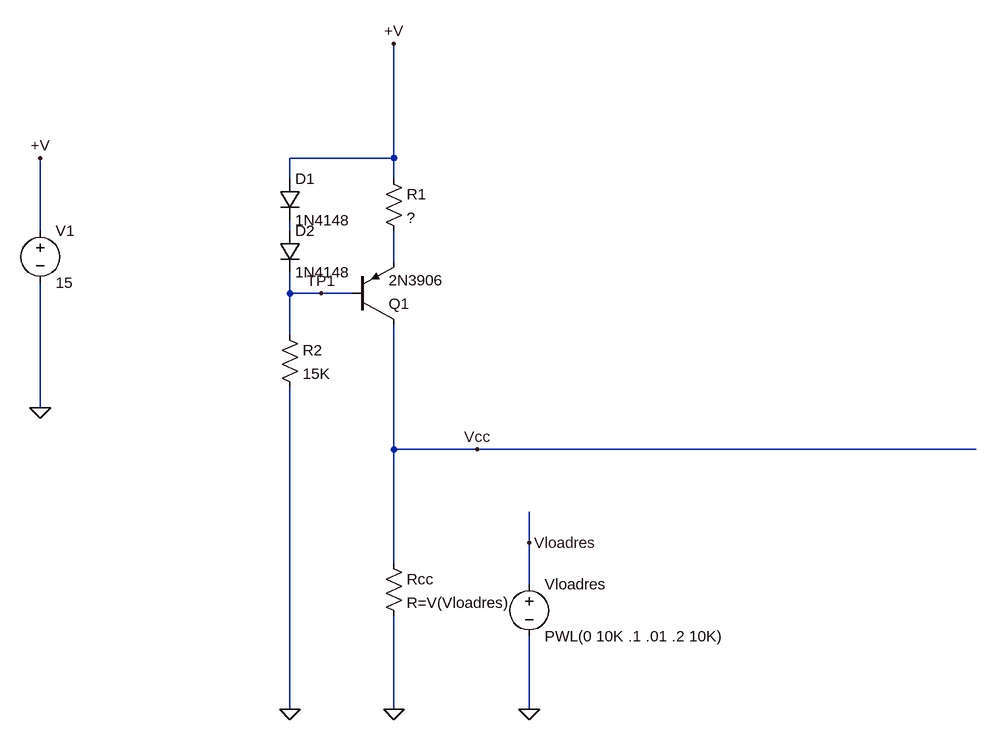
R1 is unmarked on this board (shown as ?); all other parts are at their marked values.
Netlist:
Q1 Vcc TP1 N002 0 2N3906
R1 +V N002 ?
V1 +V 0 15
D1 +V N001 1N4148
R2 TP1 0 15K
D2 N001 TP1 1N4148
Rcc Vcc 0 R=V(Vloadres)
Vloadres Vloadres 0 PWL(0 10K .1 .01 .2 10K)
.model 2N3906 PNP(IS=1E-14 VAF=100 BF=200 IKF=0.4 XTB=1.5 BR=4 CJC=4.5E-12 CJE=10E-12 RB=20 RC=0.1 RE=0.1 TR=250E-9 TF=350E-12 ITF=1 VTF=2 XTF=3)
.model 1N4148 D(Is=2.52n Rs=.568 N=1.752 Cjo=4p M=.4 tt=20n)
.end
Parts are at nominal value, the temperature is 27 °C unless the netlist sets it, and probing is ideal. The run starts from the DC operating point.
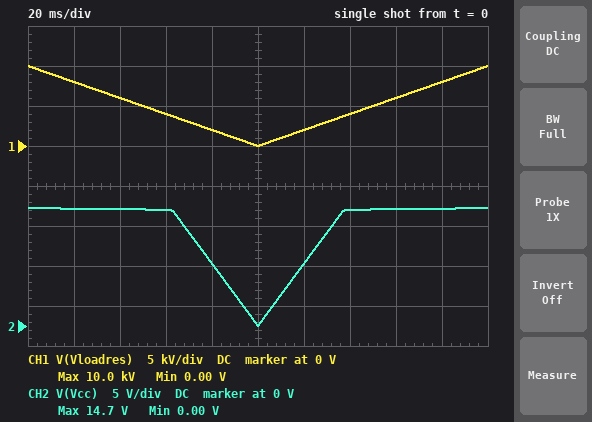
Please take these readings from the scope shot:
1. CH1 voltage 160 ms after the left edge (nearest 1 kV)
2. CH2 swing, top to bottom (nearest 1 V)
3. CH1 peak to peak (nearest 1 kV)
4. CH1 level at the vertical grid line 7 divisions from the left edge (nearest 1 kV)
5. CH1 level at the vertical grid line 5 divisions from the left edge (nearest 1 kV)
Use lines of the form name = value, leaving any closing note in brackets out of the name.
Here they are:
CH1 voltage 160 ms after the left edge = 6 kV
CH2 swing, top to bottom = 15 V
CH1 peak to peak = 10 kV
CH1 level at the vertical grid line 7 divisions from the left edge = 4 kV
CH1 level at the vertical grid line 5 divisions from the left edge = 0 V
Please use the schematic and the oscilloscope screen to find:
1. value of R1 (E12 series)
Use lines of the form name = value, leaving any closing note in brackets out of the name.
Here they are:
value of R1 = 120 Ω
